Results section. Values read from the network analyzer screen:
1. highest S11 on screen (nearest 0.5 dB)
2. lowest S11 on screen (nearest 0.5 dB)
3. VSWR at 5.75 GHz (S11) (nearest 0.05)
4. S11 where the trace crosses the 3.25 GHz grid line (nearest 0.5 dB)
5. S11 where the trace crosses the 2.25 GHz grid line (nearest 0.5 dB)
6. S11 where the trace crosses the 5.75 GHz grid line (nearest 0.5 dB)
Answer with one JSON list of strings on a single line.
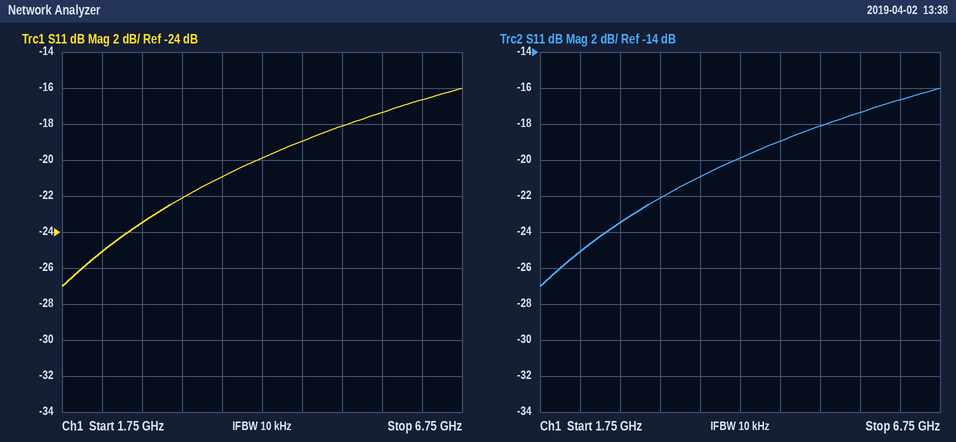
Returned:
["-16.0 dB", "-27.0 dB", "1.30", "-22.0 dB", "-25.0 dB", "-17.5 dB"]
